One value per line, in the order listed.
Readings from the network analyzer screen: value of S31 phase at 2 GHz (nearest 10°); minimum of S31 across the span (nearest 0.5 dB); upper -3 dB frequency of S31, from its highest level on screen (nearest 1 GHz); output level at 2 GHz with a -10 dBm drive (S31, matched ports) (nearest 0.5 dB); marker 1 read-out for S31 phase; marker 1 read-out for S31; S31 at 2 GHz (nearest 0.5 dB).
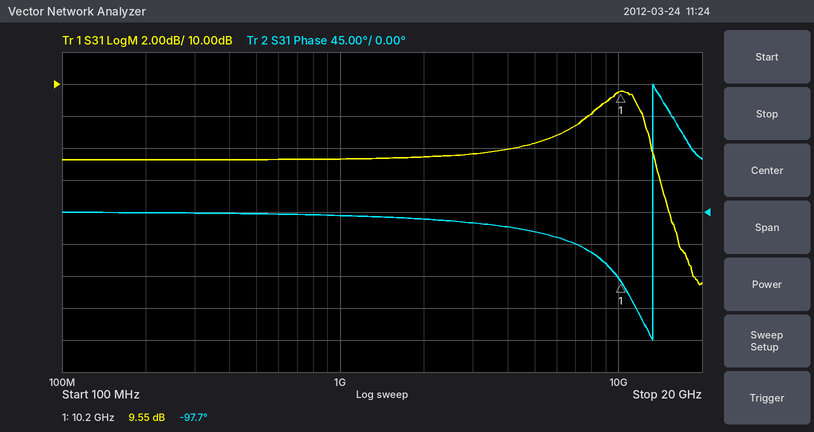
-10°
-2.5 dB
13 GHz
-4.5 dBm
-97.7°
9.55 dB
5.5 dB
